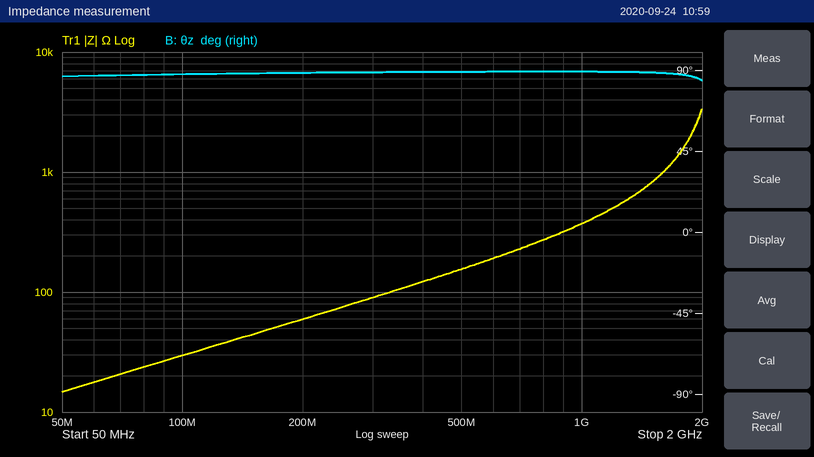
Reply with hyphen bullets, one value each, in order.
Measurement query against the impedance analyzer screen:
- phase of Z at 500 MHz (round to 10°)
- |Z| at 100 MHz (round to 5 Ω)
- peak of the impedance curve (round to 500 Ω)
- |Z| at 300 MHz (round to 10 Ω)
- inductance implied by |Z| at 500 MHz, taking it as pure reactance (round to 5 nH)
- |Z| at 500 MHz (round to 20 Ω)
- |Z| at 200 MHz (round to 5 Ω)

- 90°
- 30 Ω
- 3.5 kΩ
- 90 Ω
- 50 nH
- 160 Ω
- 60 Ω
